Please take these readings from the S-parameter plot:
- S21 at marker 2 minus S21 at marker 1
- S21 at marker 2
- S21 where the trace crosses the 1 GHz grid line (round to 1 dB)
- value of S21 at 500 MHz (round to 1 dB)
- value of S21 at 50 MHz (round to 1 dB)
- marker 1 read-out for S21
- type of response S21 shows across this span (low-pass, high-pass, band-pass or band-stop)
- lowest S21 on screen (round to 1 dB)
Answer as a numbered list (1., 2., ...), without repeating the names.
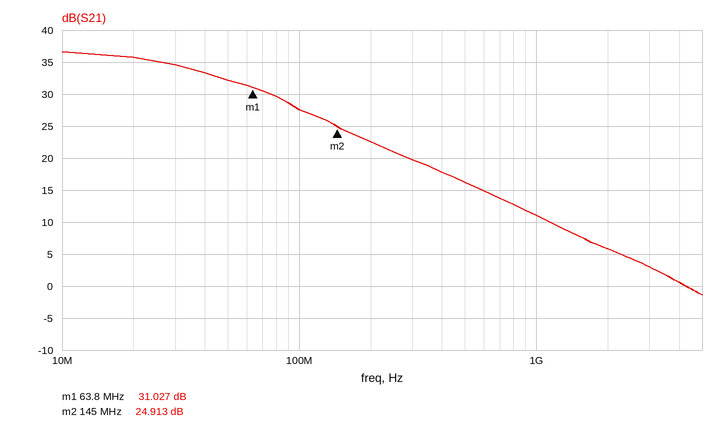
1. -6.114 dB
2. 24.913 dB
3. 11 dB
4. 16 dB
5. 32 dB
6. 31.027 dB
7. low-pass
8. -1 dB
